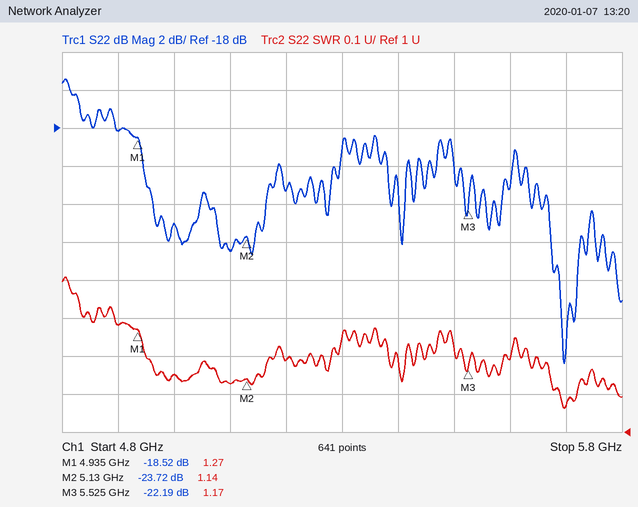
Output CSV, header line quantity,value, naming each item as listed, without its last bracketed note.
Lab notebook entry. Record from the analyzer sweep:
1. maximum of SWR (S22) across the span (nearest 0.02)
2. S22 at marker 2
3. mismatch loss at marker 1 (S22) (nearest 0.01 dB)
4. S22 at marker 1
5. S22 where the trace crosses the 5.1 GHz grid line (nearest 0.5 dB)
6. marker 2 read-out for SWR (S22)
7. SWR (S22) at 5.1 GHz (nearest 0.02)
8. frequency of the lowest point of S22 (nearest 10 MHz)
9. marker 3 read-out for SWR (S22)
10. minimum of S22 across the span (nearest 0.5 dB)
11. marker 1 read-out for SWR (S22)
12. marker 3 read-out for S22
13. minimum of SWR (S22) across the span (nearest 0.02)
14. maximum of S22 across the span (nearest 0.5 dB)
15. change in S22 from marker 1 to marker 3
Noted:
quantity,value
maximum of SWR (S22) across the span,1.40
S22 at marker 2,-23.72 dB
mismatch loss at marker 1 (S22),0.06 dB
S22 at marker 1,-18.52 dB
S22 where the trace crosses the 5.1 GHz grid line,-24.5 dB
marker 2 read-out for SWR,1.14
SWR (S22) at 5.1 GHz,1.12
frequency of the lowest point of S22,5.70 GHz
marker 3 read-out for SWR,1.17
minimum of S22 across the span,-30.5 dB
marker 1 read-out for SWR,1.27
marker 3 read-out for S22,-22.19 dB
minimum of SWR (S22) across the span,1.06
maximum of S22 across the span,-15.5 dB
change in S22 from marker 1 to marker 3,-3.67 dB
